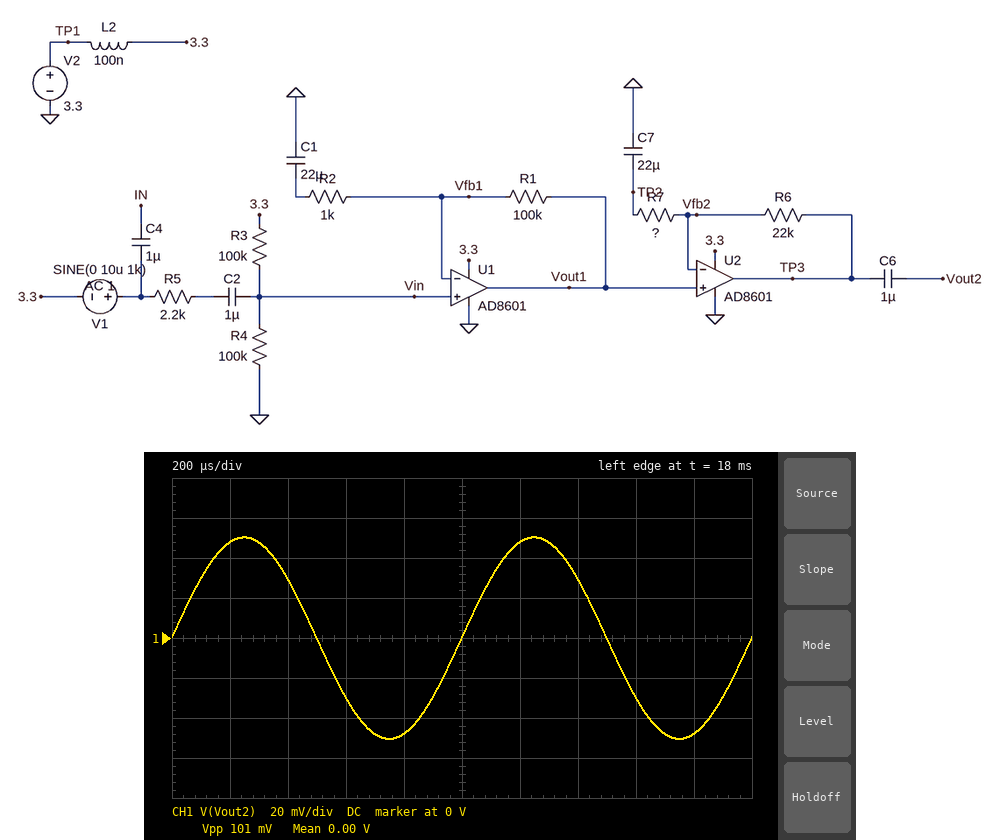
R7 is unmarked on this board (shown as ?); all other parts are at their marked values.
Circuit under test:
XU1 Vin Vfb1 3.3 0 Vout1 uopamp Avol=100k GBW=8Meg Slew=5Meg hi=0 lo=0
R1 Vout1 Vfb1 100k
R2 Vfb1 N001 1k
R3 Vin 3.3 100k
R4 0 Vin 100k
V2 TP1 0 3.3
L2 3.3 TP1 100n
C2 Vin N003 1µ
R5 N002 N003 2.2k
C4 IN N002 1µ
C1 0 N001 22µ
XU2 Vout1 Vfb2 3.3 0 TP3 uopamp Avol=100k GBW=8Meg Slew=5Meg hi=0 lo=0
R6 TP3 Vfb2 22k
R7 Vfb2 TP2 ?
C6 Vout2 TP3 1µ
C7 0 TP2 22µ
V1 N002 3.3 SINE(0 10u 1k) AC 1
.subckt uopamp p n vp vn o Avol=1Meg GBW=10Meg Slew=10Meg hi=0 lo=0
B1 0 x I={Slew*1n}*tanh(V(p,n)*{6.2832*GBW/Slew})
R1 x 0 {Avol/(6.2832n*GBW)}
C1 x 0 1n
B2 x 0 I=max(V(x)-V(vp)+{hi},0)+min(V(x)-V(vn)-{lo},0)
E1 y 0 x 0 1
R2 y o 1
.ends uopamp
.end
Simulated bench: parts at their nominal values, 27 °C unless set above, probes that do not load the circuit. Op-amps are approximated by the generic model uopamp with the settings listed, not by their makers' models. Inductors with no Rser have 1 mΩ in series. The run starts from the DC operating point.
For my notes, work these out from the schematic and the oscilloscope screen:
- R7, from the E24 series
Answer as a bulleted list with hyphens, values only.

- 430 Ω
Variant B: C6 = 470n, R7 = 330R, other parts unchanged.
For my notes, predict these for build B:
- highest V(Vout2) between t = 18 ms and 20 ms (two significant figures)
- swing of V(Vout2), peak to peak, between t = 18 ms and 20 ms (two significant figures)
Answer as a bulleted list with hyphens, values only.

- 65 mV
- 130 mV
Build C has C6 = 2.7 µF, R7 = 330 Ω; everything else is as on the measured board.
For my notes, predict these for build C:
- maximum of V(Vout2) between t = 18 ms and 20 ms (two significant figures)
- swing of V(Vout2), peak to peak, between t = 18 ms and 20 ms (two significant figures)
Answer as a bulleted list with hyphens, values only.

- 65 mV
- 130 mV
